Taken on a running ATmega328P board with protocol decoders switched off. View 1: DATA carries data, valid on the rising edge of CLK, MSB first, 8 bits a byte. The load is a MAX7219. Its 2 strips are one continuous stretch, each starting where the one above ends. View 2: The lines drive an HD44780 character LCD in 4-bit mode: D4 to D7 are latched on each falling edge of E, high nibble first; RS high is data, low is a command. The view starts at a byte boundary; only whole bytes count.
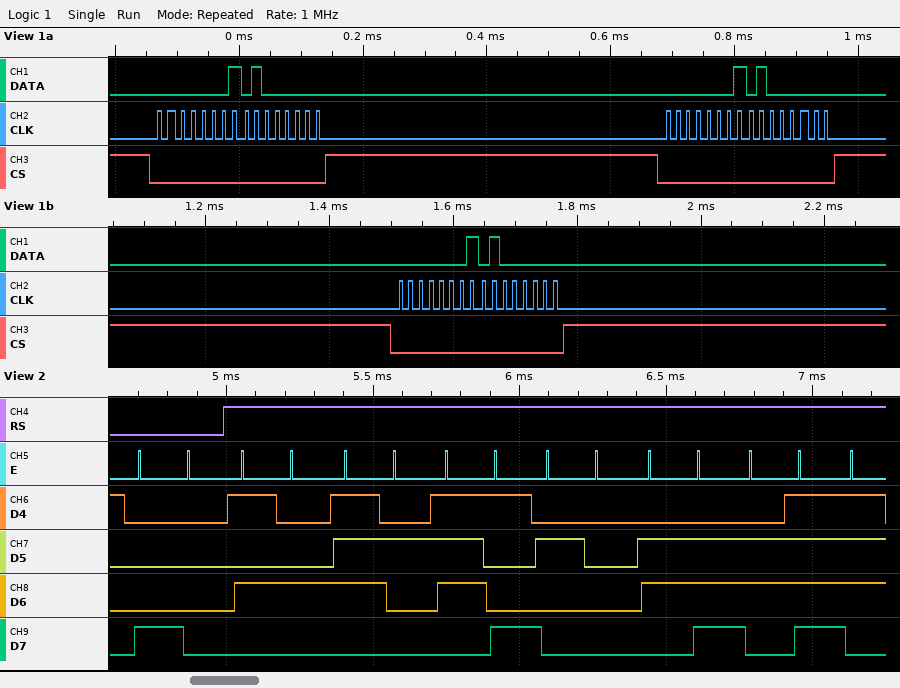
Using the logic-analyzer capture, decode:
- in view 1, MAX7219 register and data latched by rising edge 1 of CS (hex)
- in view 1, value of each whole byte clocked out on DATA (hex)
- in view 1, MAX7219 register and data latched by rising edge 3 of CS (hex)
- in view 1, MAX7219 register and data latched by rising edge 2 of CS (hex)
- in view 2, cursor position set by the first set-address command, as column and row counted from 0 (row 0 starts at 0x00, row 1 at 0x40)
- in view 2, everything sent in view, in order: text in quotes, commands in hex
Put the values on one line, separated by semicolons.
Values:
register 0x1, data 0x40; 01 40 01 40 01 40; register 0x1, data 0x40; register 0x1, data 0x40; column 0, row 0; 0x80 "Try no"
